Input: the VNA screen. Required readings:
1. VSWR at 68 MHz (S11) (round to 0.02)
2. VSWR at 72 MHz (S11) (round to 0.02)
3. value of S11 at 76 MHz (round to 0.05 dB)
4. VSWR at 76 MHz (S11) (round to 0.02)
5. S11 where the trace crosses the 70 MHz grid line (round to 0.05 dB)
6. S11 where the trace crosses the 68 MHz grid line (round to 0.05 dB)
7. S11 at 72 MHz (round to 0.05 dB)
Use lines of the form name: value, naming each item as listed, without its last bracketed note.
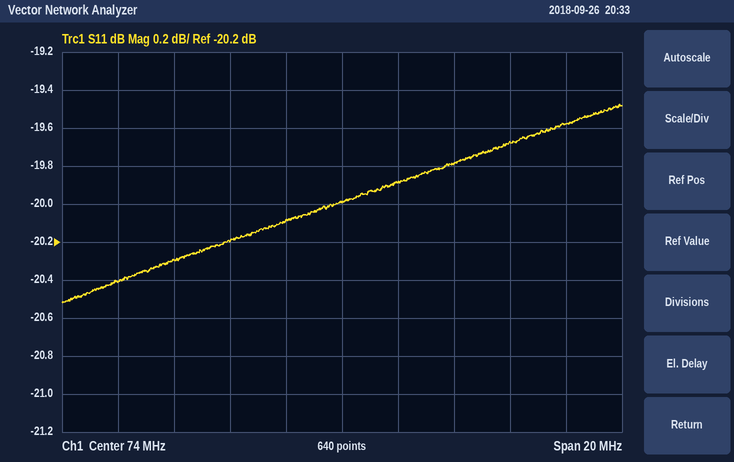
VSWR at 68 MHz (S11): 1.22
VSWR at 72 MHz (S11): 1.22
value of S11 at 76 MHz: -19.90 dB
VSWR at 76 MHz (S11): 1.22
S11 where the trace crosses the 70 MHz grid line: -20.20 dB
S11 where the trace crosses the 68 MHz grid line: -20.30 dB
S11 at 72 MHz: -20.10 dB
